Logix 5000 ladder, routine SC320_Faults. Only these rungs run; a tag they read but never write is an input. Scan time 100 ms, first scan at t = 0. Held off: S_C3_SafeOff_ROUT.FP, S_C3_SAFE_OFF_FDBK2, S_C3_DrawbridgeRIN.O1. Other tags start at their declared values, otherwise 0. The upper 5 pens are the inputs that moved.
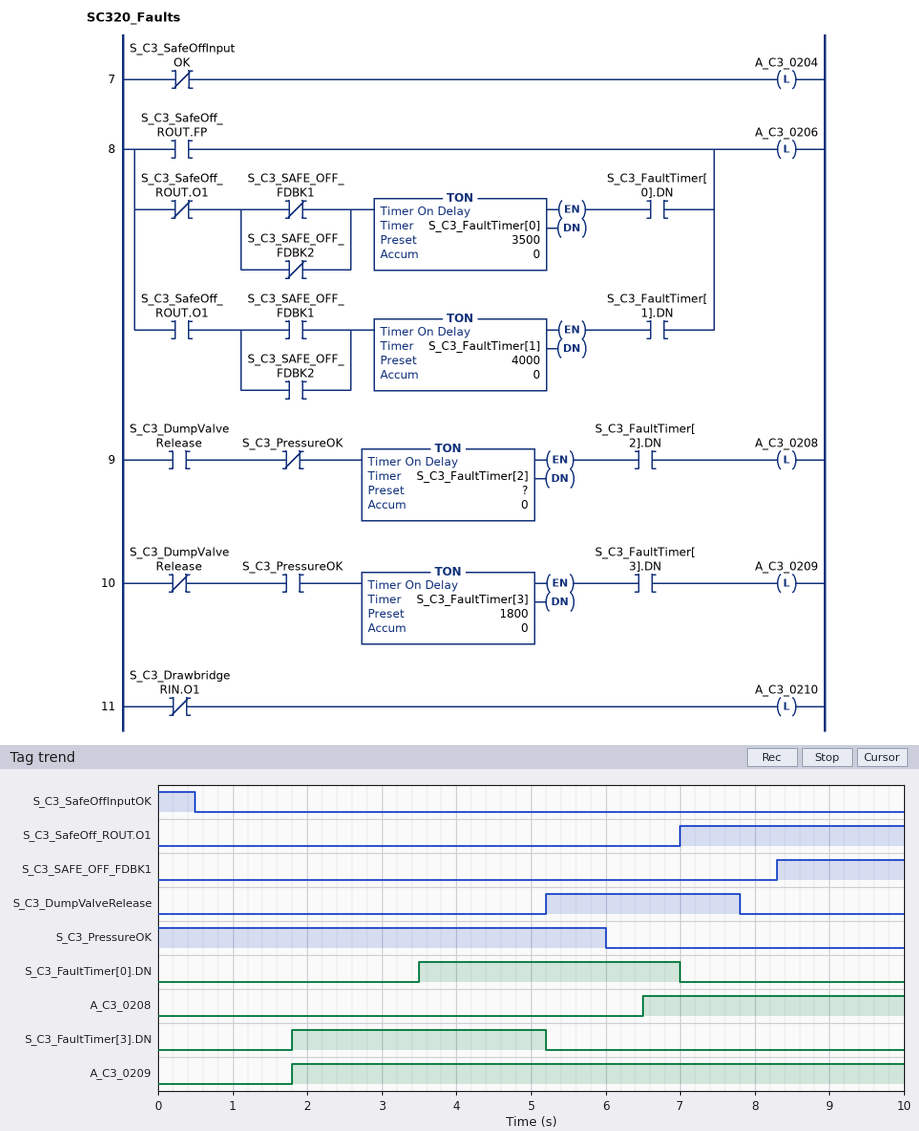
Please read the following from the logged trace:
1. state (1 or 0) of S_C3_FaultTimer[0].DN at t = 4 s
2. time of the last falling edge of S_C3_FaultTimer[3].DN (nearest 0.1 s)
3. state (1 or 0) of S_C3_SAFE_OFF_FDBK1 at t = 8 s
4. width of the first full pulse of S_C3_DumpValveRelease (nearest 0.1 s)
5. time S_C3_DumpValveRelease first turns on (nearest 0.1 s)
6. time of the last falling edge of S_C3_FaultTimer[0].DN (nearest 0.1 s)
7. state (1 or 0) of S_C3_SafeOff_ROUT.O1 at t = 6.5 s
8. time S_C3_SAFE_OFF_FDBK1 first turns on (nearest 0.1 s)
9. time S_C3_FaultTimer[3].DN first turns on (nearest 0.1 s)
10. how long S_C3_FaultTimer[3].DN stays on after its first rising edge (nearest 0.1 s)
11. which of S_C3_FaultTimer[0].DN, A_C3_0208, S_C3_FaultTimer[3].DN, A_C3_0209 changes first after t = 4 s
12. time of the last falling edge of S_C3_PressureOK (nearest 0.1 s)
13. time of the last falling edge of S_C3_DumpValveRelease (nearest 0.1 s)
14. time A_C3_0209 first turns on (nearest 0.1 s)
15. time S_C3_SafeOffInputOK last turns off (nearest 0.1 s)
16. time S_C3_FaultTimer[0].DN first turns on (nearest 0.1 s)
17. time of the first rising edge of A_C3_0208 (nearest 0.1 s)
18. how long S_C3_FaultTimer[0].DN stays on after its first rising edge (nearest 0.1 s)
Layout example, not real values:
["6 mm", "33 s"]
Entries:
["1", "5.2 s", "0", "2.6 s", "5.2 s", "7.0 s", "0", "8.3 s", "1.8 s", "3.4 s", "S_C3_FaultTimer[3].DN", "6.0 s", "7.8 s", "1.8 s", "0.5 s", "3.5 s", "6.5 s", "3.5 s"]
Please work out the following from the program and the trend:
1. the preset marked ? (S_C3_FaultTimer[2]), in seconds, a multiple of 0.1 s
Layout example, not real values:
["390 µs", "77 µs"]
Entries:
["0.5 s"]
